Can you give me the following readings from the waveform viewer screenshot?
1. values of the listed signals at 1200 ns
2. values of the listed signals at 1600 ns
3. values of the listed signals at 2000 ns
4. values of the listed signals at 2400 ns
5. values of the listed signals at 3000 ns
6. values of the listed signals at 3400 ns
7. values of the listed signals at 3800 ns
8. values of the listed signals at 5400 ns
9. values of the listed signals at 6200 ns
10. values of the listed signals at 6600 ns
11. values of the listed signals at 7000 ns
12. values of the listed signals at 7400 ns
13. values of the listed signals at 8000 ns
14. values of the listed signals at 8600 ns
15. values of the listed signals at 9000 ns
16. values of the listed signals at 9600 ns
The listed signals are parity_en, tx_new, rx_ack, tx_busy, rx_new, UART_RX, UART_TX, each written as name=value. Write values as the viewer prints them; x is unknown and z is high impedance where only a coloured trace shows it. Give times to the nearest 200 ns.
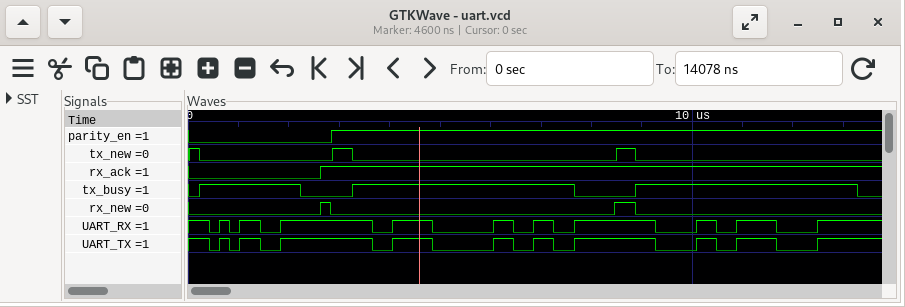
parity_en=0, tx_new=0, rx_ack=0, tx_busy=1, rx_new=0, UART_RX=1, UART_TX=1
parity_en=0, tx_new=0, rx_ack=0, tx_busy=1, rx_new=0, UART_RX=0, UART_TX=0
parity_en=0, tx_new=0, rx_ack=0, tx_busy=1, rx_new=0, UART_RX=1, UART_TX=1
parity_en=0, tx_new=0, rx_ack=0, tx_busy=0, rx_new=0, UART_RX=1, UART_TX=1
parity_en=1, tx_new=1, rx_ack=1, tx_busy=0, rx_new=0, UART_RX=1, UART_TX=1
parity_en=1, tx_new=0, rx_ack=1, tx_busy=1, rx_new=0, UART_RX=1, UART_TX=1
parity_en=1, tx_new=0, rx_ack=1, tx_busy=1, rx_new=0, UART_RX=0, UART_TX=0
parity_en=1, tx_new=0, rx_ack=1, tx_busy=1, rx_new=0, UART_RX=0, UART_TX=0
parity_en=1, tx_new=0, rx_ack=1, tx_busy=1, rx_new=0, UART_RX=1, UART_TX=1
parity_en=1, tx_new=0, rx_ack=1, tx_busy=1, rx_new=0, UART_RX=0, UART_TX=0
parity_en=1, tx_new=0, rx_ack=1, tx_busy=1, rx_new=0, UART_RX=1, UART_TX=1
parity_en=1, tx_new=0, rx_ack=1, tx_busy=1, rx_new=0, UART_RX=0, UART_TX=0
parity_en=1, tx_new=0, rx_ack=1, tx_busy=0, rx_new=0, UART_RX=1, UART_TX=1
parity_en=1, tx_new=1, rx_ack=1, tx_busy=0, rx_new=1, UART_RX=1, UART_TX=1
parity_en=1, tx_new=0, rx_ack=1, tx_busy=1, rx_new=0, UART_RX=1, UART_TX=1
parity_en=1, tx_new=0, rx_ack=1, tx_busy=1, rx_new=0, UART_RX=0, UART_TX=0
